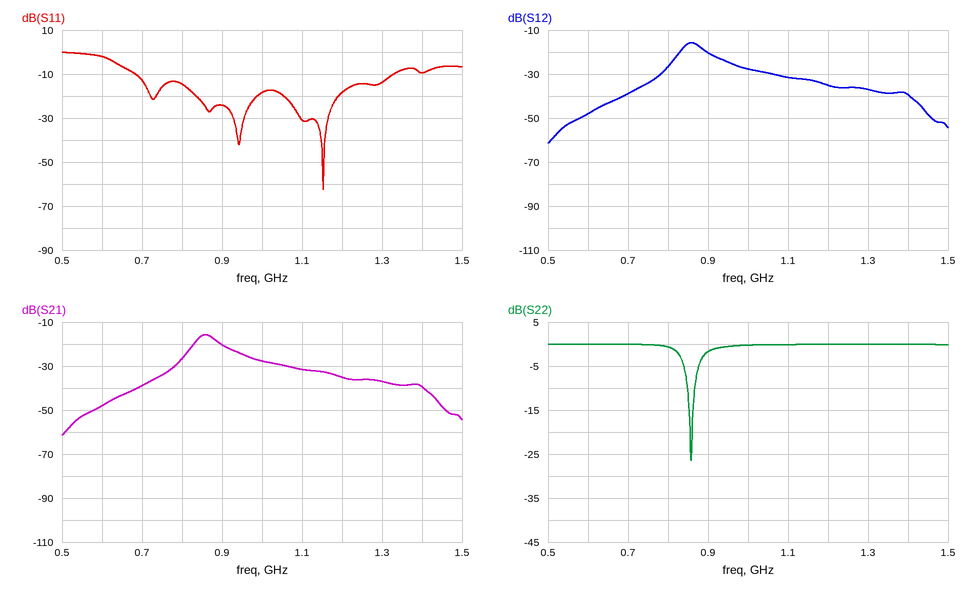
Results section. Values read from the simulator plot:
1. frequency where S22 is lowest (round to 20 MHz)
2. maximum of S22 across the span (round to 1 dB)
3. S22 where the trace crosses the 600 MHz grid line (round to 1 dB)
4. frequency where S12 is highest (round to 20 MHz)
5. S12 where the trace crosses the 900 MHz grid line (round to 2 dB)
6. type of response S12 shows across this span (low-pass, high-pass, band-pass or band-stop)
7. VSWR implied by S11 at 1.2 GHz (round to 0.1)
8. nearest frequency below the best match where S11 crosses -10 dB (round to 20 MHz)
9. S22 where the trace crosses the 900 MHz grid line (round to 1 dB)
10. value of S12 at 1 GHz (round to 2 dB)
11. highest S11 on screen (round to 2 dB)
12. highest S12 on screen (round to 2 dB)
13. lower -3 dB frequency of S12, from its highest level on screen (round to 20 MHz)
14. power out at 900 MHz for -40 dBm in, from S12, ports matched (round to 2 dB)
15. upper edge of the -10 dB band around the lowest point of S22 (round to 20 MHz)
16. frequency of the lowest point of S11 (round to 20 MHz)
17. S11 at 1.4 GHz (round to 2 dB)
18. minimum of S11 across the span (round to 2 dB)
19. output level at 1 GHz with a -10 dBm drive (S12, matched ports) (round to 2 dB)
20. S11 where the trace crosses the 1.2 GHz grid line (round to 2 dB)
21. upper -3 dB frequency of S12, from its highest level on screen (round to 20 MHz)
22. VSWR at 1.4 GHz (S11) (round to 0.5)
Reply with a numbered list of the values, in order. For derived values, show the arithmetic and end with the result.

1. 860 MHz
2. 0 dB
3. 0 dB
4. 860 MHz
5. -20 dB
6. band-pass
7. |Γ| = 10^(-18/20) = 0.1259; VSWR = (1 + 0.1259)/(1 − 0.1259) ≈ 1.3
8. 680 MHz
9. -2 dB
10. -28 dB
11. 0 dB
12. -16 dB
13. 840 MHz
14. -40 dBm + (-20 dB) = -60 dBm
15. 860 MHz
16. 1.16 GHz
17. -10 dB
18. -62 dB
19. -10 dBm + (-28 dB) = -38 dBm
20. -18 dB
21. 880 MHz
22. |Γ| = 10^(-10/20) = 0.3162; VSWR = (1 + 0.3162)/(1 − 0.3162) ≈ 1.92, so 2.0 to the nearest 0.5
